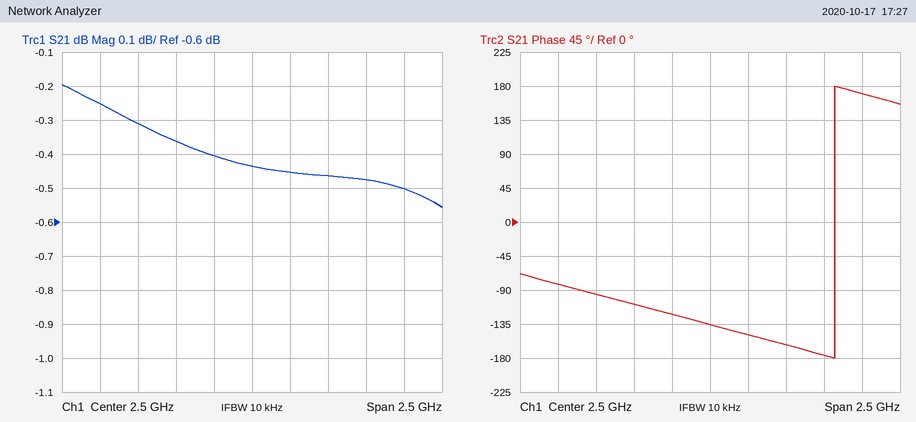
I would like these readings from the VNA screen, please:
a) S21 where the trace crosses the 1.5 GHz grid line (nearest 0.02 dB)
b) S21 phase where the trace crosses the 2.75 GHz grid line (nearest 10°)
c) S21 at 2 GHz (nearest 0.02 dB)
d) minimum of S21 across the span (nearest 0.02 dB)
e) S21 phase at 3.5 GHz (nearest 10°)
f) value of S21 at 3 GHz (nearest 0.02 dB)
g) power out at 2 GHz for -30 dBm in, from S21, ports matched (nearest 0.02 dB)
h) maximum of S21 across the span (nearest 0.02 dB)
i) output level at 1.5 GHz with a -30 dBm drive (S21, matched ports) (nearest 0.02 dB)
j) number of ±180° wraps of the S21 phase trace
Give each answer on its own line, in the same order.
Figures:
-0.26 dB
-150°
-0.36 dB
-0.56 dB
170°
-0.46 dB
-30.36 dBm
-0.20 dB
-30.26 dBm
1
